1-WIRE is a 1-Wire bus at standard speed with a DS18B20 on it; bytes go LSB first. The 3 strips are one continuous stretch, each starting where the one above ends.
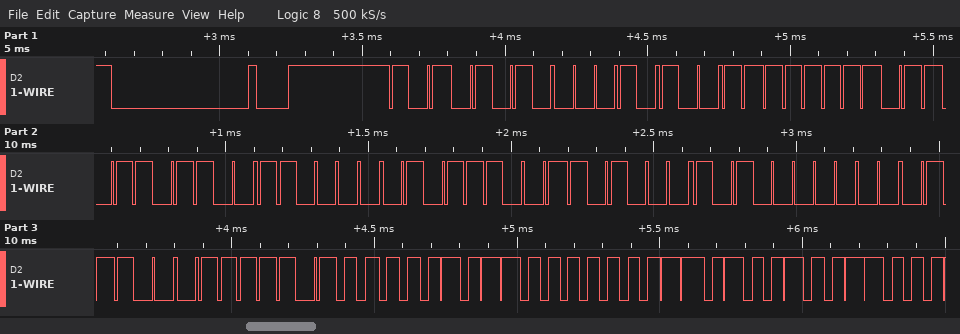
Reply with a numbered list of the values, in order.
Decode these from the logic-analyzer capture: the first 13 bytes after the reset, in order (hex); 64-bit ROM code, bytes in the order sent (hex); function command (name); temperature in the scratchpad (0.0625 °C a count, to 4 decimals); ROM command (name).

1. 55 28 FF B6 19 74 16 05 38 BE A0 01 4B
2. 28 FF B6 19 74 16 05 38
3. Read Scratchpad
4. 26.0000 °C
5. Match ROM
